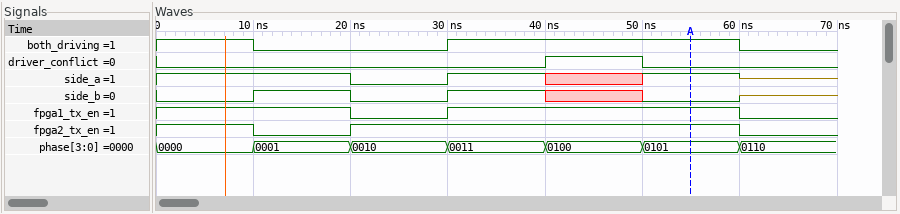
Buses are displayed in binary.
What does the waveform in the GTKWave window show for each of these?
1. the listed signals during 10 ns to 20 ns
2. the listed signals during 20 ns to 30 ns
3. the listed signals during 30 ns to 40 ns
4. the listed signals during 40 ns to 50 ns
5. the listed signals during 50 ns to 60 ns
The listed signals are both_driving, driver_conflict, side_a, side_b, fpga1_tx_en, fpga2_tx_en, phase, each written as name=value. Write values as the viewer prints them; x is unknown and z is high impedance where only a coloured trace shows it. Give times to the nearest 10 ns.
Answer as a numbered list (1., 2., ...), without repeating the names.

1. both_driving=0, driver_conflict=0, side_a=1, side_b=1, fpga1_tx_en=1, fpga2_tx_en=0, phase=0001
2. both_driving=0, driver_conflict=0, side_a=0, side_b=0, fpga1_tx_en=0, fpga2_tx_en=1, phase=0010
3. both_driving=1, driver_conflict=0, side_a=1, side_b=1, fpga1_tx_en=1, fpga2_tx_en=1, phase=0011
4. both_driving=1, driver_conflict=1, side_a=x, side_b=x, fpga1_tx_en=1, fpga2_tx_en=1, phase=0100
5. both_driving=1, driver_conflict=0, side_a=1, side_b=0, fpga1_tx_en=1, fpga2_tx_en=1, phase=0101
